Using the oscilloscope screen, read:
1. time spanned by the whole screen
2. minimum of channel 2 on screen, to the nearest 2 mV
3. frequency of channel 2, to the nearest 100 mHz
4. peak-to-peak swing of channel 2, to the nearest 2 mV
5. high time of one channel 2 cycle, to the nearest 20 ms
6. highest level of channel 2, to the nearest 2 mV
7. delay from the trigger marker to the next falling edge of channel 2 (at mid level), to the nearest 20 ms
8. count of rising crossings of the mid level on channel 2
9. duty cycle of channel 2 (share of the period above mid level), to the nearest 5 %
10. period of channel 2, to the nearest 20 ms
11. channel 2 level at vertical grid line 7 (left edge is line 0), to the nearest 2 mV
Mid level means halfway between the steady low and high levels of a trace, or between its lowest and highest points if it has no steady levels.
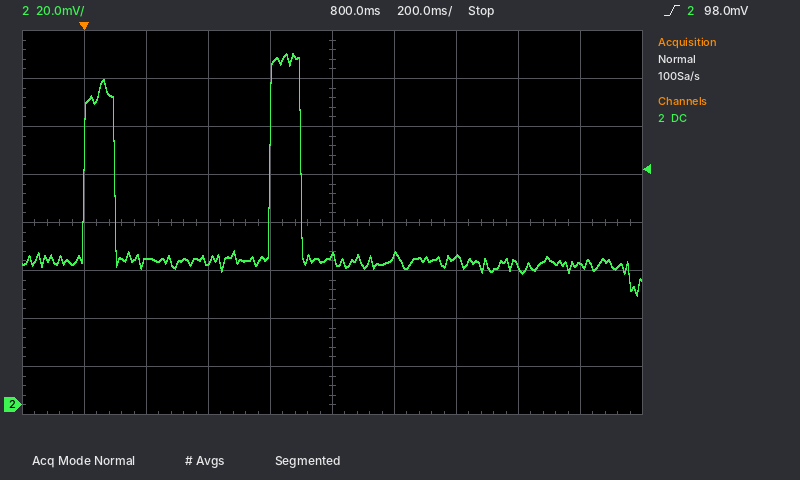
2 s
46 mV
1.7 Hz
100 mV
100 ms
146 mV
100 ms
2
15 %
600 ms
62 mV
